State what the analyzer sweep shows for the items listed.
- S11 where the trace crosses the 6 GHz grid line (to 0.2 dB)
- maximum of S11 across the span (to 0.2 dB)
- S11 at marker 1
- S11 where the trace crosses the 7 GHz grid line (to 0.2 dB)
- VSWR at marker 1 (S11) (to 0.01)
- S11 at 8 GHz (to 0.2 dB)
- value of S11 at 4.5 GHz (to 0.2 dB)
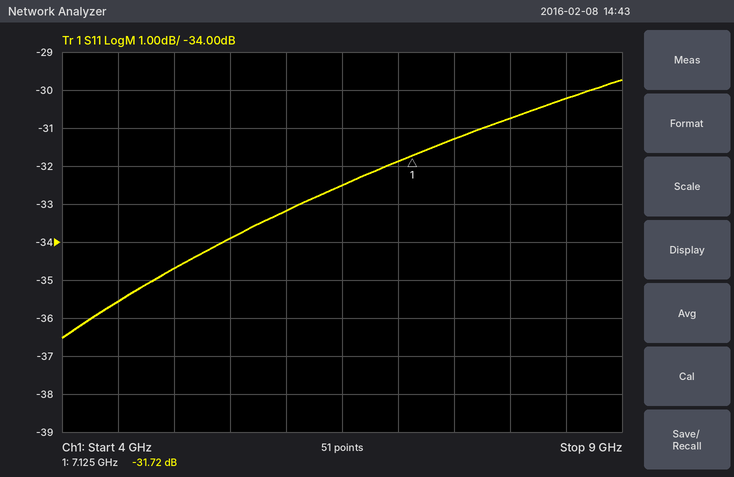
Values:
-33.2 dB
-29.8 dB
-31.72 dB
-31.8 dB
1.05
-30.8 dB
-35.6 dB
